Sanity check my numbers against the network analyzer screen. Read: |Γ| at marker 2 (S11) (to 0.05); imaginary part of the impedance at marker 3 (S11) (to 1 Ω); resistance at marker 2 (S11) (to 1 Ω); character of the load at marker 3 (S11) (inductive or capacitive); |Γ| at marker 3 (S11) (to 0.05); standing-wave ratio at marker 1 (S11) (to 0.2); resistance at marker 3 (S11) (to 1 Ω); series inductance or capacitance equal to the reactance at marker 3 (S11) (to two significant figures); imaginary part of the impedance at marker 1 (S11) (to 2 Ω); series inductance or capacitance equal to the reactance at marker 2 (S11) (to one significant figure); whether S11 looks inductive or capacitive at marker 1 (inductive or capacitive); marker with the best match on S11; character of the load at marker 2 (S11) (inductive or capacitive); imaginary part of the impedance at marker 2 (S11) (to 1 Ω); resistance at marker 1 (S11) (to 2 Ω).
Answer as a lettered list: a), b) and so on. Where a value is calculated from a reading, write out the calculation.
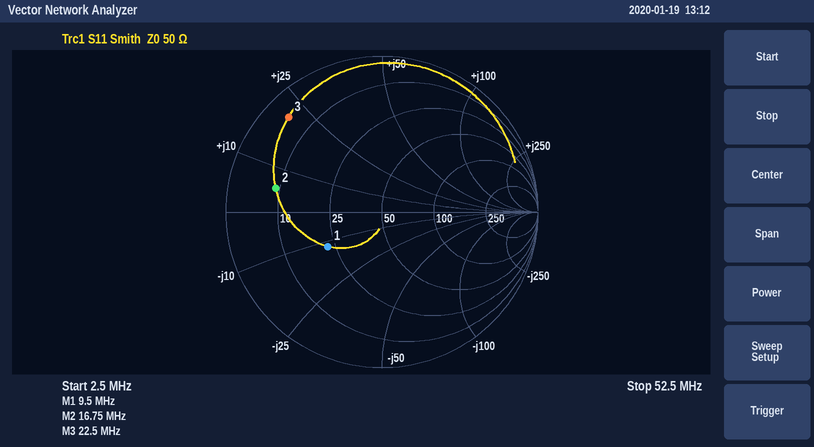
a) 0.70
b) +21 Ω
c) 9 Ω
d) inductive
e) 0.85
f) 2.4
g) 5 Ω
h) L = 21 Ω/(2π × 22.5 MHz) ≈ 149 nH, so 150 nH to two significant figures
i) -12 Ω
j) L = 5 Ω/(2π × 16.75 MHz) ≈ 47.5 nH, so 50 nH to one significant figure
k) capacitive
l) marker 1
m) inductive
n) +5 Ω
o) 22 Ω
